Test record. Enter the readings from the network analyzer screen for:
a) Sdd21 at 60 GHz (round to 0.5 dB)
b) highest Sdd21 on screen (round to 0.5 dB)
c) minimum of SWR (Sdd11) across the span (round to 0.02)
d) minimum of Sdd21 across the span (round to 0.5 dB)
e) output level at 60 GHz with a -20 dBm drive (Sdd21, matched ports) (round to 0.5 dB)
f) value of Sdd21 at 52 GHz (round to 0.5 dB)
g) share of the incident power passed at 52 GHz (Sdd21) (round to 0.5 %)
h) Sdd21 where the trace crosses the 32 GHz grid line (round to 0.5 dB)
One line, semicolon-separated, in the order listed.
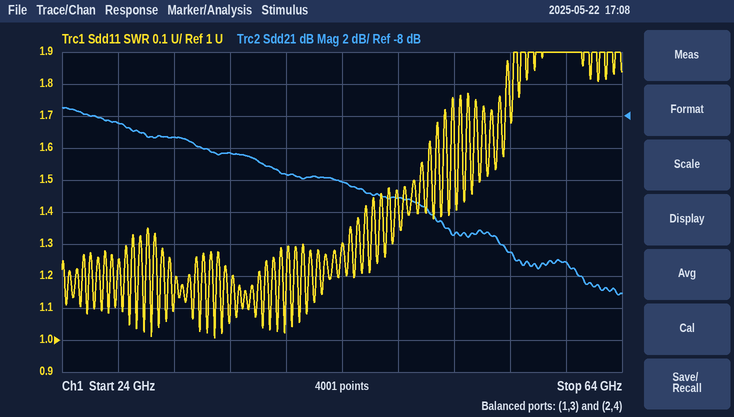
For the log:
-17.0 dB; -7.5 dB; 1.00; -19.0 dB; -37.0 dBm; -15.5 dB; 3.0 %; -9.5 dB
